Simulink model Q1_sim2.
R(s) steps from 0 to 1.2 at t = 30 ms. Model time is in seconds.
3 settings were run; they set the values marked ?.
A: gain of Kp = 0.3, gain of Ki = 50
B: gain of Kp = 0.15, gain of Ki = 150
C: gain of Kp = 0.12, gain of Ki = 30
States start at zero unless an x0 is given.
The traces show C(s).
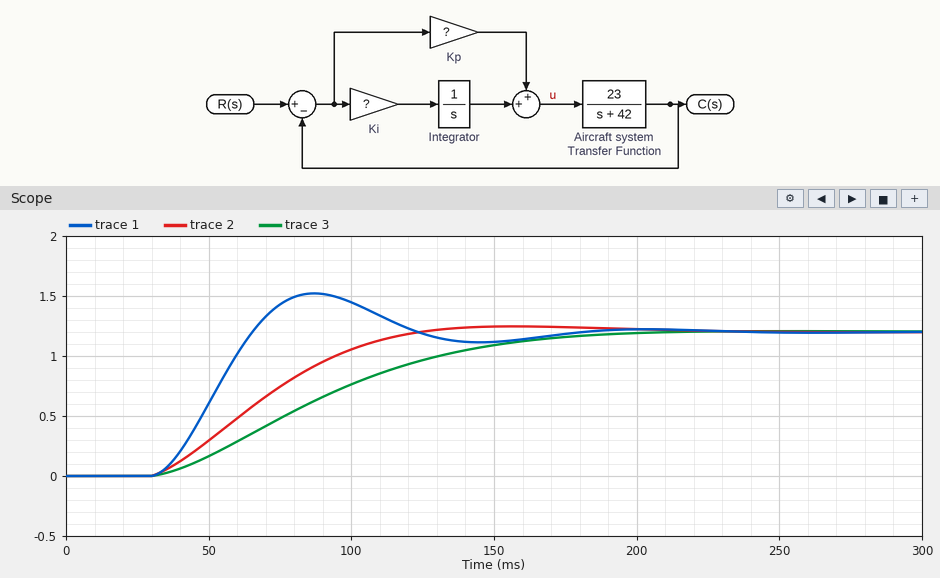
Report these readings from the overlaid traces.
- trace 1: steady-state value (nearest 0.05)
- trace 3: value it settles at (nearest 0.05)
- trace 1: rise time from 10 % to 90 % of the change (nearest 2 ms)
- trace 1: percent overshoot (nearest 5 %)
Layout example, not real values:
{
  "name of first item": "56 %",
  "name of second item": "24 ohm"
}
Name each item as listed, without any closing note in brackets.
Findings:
{
  "trace 1: steady-state value": "1.20",
  "trace 3: value it settles at": "1.20",
  "trace 1: rise time from 10 % to 90 % of the change": "24 ms",
  "trace 1: percent overshoot": "25 %"
}
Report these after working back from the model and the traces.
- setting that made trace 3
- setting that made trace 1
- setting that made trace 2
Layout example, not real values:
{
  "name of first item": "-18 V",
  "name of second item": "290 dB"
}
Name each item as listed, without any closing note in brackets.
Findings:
{
  "setting that made trace 3": "C",
  "setting that made trace 1": "B",
  "setting that made trace 2": "A"
}
